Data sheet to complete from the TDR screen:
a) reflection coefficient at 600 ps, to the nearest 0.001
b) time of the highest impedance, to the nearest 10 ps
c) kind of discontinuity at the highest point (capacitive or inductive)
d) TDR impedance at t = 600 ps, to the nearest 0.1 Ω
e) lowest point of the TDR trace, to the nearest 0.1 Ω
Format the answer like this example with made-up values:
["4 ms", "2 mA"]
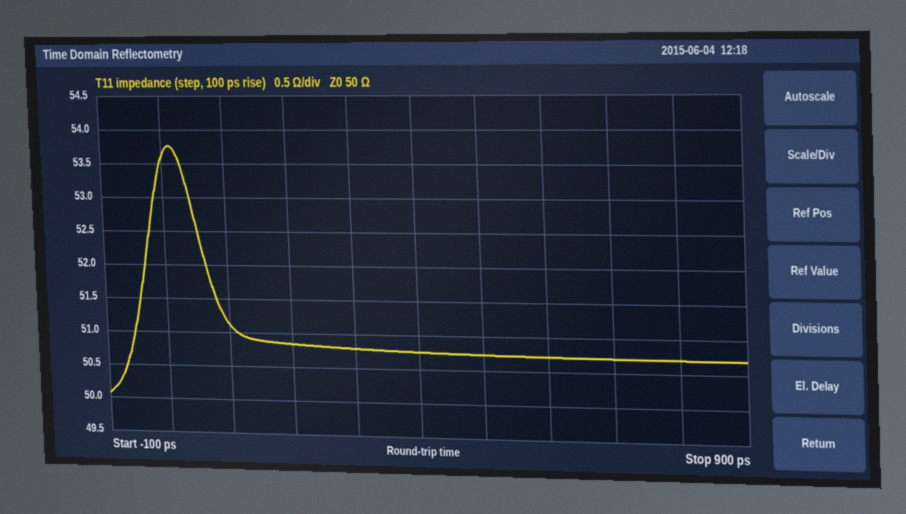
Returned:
["+0.007", "10 ps", "inductive", "50.7 Ω", "50.1 Ω"]
